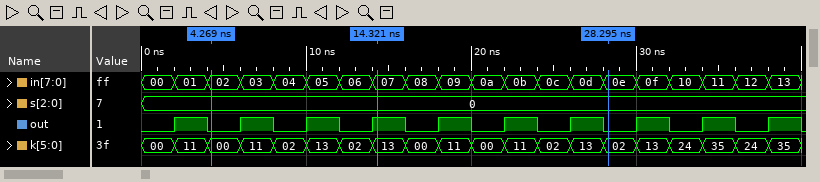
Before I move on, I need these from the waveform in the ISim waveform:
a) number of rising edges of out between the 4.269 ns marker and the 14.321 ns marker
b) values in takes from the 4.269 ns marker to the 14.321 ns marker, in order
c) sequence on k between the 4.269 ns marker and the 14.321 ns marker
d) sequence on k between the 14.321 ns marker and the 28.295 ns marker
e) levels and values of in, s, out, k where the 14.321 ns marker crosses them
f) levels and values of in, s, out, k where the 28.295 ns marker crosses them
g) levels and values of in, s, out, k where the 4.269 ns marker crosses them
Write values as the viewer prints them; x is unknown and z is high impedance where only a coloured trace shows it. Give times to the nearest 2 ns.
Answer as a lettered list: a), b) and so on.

a) 3
b) 02, 03, 04, 05, 06, 07
c) 00, 11, 02, 13, 02, 13
d) 13, 00, 11, 00, 11, 02, 13, 02
e) in=07, s=0, out=1, k=13
f) in=0e, s=0, out=0, k=02
g) in=02, s=0, out=0, k=00
